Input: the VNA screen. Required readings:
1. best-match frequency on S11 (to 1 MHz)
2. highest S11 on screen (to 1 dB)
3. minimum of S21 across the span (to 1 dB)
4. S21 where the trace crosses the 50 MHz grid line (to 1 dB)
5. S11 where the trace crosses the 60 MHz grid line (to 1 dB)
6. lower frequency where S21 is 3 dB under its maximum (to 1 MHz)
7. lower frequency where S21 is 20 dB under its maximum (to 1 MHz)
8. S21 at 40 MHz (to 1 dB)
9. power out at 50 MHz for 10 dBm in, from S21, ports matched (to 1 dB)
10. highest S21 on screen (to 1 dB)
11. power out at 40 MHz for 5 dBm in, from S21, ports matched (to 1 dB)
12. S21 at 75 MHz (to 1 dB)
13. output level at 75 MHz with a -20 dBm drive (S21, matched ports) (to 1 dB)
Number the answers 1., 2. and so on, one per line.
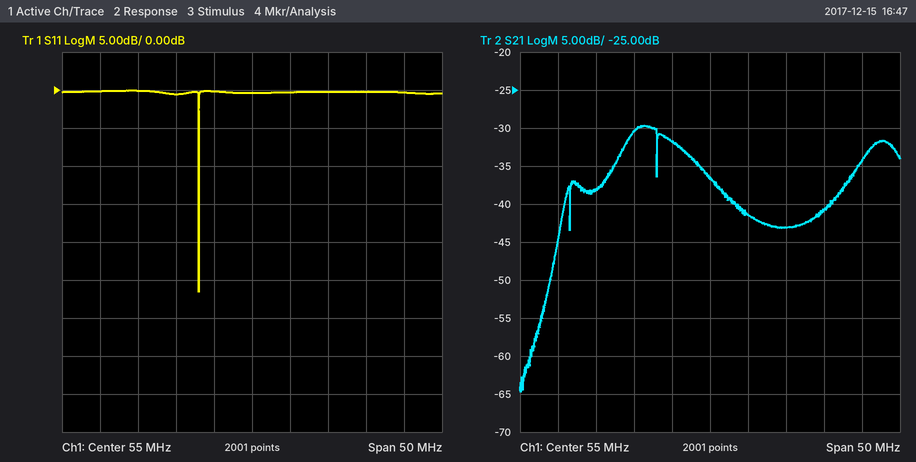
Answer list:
1. 48 MHz
2. 0 dB
3. -65 dB
4. -32 dB
5. 0 dB
6. 44 MHz
7. 34 MHz
8. -38 dB
9. -22 dBm
10. -30 dB
11. -33 dBm
12. -34 dB
13. -54 dBm
